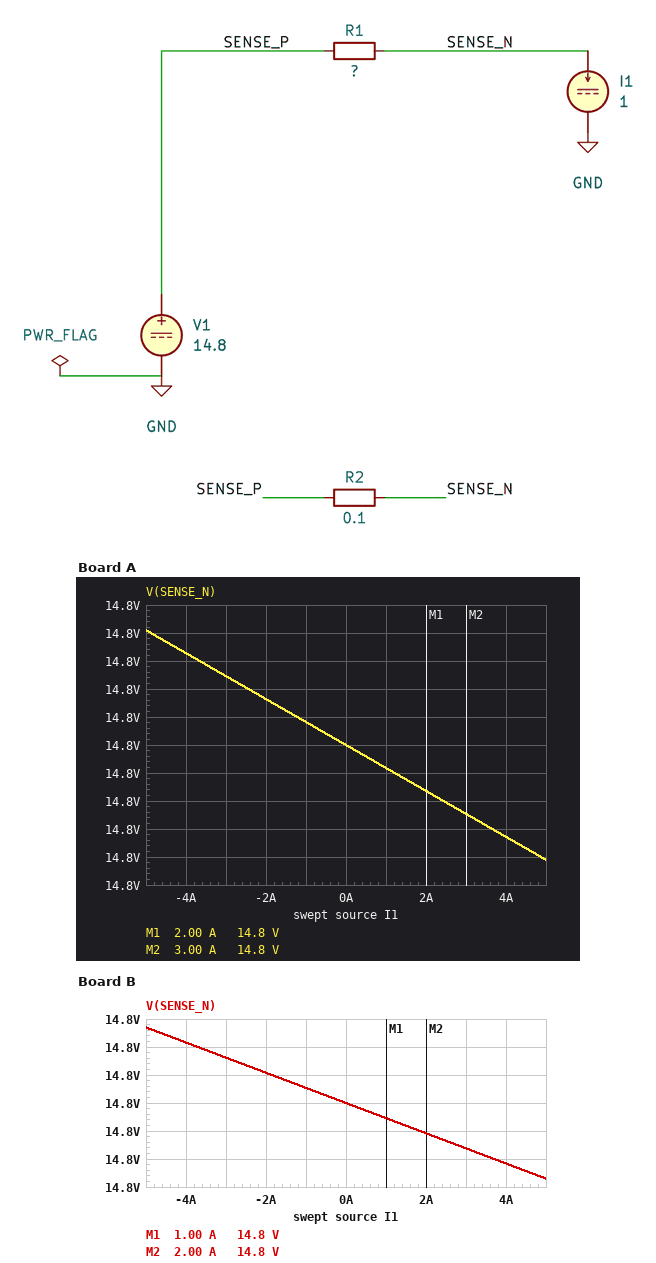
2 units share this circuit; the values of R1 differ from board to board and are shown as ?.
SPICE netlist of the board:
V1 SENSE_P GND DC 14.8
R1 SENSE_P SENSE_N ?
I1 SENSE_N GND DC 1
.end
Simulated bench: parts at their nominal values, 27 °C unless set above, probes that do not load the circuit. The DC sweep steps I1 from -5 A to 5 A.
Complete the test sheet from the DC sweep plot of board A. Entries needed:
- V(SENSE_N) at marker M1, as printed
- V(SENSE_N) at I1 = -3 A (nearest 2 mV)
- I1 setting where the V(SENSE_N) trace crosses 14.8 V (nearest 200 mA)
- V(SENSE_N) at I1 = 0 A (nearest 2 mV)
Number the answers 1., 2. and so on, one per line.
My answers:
1. 14.8 V
2. 14.824 V
3. 2.4 A
4. 14.800 V
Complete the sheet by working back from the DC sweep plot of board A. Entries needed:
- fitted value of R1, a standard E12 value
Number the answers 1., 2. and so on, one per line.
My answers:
1. 8.2 mΩ
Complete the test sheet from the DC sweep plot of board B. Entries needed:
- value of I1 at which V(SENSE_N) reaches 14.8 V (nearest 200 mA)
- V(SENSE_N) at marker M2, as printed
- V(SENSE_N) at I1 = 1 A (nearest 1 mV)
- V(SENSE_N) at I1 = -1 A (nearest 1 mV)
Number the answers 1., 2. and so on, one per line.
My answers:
1. 0 A
2. 14.8 V
3. 14.797 V
4. 14.803 V
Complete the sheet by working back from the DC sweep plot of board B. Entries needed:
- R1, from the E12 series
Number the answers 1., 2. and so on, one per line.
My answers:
1. 2.7 mΩ
